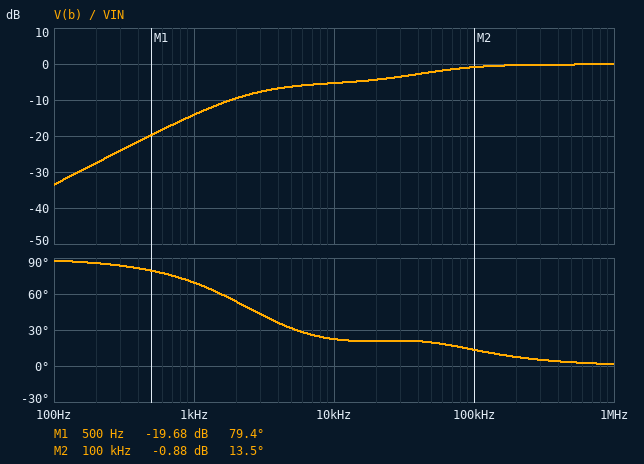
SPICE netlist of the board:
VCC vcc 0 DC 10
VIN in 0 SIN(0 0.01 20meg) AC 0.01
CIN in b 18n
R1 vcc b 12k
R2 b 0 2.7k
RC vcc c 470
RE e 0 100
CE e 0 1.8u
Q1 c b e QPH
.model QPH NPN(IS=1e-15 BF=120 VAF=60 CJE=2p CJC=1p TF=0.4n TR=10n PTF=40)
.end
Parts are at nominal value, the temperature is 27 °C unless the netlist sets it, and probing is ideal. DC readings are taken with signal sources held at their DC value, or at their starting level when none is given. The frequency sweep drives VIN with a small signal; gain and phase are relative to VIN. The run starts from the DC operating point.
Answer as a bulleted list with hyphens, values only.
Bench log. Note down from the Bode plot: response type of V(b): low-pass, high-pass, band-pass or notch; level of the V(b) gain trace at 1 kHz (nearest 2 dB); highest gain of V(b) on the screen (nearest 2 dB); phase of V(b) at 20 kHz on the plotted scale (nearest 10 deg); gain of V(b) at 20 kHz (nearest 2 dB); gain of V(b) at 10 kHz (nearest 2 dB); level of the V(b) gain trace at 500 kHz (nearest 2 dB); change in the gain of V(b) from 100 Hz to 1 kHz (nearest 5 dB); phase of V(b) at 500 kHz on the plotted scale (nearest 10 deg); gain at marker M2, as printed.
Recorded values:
- high-pass
- -14 dB
- 0 dB
- 20 deg
- -4 dB
- -6 dB
- 0 dB
- 20 dB
- 0 deg
- -0.88 dB
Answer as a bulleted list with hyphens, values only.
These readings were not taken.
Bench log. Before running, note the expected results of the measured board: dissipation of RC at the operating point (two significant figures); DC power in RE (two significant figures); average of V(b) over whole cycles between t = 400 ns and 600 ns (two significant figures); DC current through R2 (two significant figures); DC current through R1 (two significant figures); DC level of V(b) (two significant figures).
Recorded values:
- 38 mW
- 8.3 mW
- 1.7 V
- 620 µA
- 690 µA
- 1.7 V
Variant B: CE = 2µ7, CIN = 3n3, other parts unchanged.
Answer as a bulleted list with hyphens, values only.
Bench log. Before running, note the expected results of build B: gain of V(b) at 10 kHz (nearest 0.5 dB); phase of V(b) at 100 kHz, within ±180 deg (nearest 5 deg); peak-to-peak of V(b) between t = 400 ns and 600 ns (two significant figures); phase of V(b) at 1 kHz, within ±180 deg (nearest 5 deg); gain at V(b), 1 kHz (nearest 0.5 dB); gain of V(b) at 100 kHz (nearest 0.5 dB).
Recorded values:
- -18.0 dB
- 50 deg
- 19 mV
- 75 deg
- -28.5 dB
- -6.0 dB
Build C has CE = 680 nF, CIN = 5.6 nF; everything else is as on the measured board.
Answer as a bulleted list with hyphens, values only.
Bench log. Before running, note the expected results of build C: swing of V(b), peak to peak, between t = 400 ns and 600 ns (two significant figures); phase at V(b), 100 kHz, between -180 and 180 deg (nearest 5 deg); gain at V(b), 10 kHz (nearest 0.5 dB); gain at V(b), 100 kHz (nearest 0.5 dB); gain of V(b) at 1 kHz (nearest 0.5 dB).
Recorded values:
- 19 mV
- 25 deg
- -8.0 dB
- -3.5 dB
- -23.5 dB
